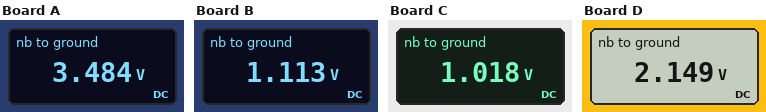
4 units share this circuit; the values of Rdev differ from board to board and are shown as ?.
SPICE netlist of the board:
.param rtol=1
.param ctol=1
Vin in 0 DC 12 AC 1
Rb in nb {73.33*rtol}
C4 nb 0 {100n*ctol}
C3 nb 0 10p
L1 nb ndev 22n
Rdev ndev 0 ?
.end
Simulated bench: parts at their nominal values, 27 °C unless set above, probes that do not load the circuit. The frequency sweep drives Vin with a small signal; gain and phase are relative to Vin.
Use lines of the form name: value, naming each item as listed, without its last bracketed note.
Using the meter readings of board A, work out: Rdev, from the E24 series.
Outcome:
Rdev, from the E24 series: 30 Ω
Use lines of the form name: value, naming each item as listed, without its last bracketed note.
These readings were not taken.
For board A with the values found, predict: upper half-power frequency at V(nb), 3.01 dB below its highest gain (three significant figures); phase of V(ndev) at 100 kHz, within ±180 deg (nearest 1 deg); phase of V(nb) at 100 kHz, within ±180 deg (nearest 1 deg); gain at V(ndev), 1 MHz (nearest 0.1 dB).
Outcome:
upper half-power frequency at V(nb), 3.01 dB below its highest gain: 74.8 kHz
phase of V(ndev) at 100 kHz, within ±180 deg: -53 deg
phase of V(nb) at 100 kHz, within ±180 deg: -53 deg
gain at V(ndev), 1 MHz: -33.3 dB
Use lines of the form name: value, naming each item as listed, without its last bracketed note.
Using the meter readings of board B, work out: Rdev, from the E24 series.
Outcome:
Rdev, from the E24 series: 7.5 Ω
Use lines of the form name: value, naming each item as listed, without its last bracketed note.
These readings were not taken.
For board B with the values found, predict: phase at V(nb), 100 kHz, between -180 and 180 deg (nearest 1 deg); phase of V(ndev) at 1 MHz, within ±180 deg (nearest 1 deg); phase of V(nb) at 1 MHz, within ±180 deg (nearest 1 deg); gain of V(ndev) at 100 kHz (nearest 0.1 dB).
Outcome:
phase at V(nb), 100 kHz, between -180 and 180 deg: -23 deg
phase of V(ndev) at 1 MHz, within ±180 deg: -78 deg
phase of V(nb) at 1 MHz, within ±180 deg: -77 deg
gain of V(ndev) at 100 kHz: -21.4 dB
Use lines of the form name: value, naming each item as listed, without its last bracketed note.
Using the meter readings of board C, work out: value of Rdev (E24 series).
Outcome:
value of Rdev: 6.8 Ω
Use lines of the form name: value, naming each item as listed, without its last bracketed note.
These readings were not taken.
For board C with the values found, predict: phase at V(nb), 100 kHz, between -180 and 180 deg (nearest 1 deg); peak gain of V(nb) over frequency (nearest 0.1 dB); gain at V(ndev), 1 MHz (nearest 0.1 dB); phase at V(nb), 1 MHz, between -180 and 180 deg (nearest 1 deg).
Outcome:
phase at V(nb), 100 kHz, between -180 and 180 deg: -21 deg
peak gain of V(nb) over frequency: -21.4 dB
gain at V(ndev), 1 MHz: -33.5 dB
phase at V(nb), 1 MHz, between -180 and 180 deg: -76 deg
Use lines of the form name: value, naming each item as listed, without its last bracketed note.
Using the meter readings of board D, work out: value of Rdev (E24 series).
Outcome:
value of Rdev: 16 Ω
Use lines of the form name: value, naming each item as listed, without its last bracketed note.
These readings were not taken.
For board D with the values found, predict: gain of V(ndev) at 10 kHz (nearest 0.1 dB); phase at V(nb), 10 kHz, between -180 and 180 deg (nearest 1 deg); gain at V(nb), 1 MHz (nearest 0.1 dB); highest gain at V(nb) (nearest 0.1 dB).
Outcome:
gain of V(ndev) at 10 kHz: -15.0 dB
phase at V(nb), 10 kHz, between -180 and 180 deg: -5 deg
gain at V(nb), 1 MHz: -33.3 dB
highest gain at V(nb): -14.9 dB
